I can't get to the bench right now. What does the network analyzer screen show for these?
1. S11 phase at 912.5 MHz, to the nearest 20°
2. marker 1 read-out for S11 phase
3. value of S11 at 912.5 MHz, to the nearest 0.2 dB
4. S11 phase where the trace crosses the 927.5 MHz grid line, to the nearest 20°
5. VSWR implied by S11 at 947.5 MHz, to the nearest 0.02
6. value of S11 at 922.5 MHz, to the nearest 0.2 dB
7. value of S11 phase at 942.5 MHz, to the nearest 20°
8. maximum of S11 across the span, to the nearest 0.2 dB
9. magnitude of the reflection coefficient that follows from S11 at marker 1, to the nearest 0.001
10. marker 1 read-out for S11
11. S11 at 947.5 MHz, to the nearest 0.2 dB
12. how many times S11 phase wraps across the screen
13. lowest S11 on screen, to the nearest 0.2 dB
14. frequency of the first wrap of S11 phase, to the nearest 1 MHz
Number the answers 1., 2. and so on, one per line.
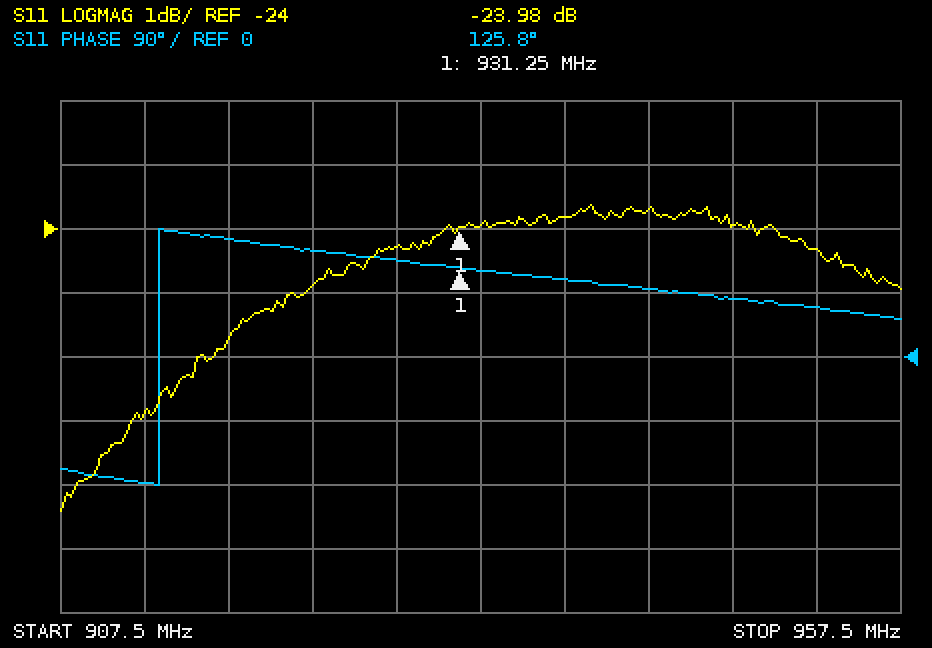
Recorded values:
1. -180°
2. 125.8°
3. -26.8 dB
4. 140°
5. 1.14
6. -24.8 dB
7. 100°
8. -23.6 dB
9. 0.063
10. -23.98 dB
11. -24.0 dB
12. 1
13. -28.4 dB
14. 913 MHz
